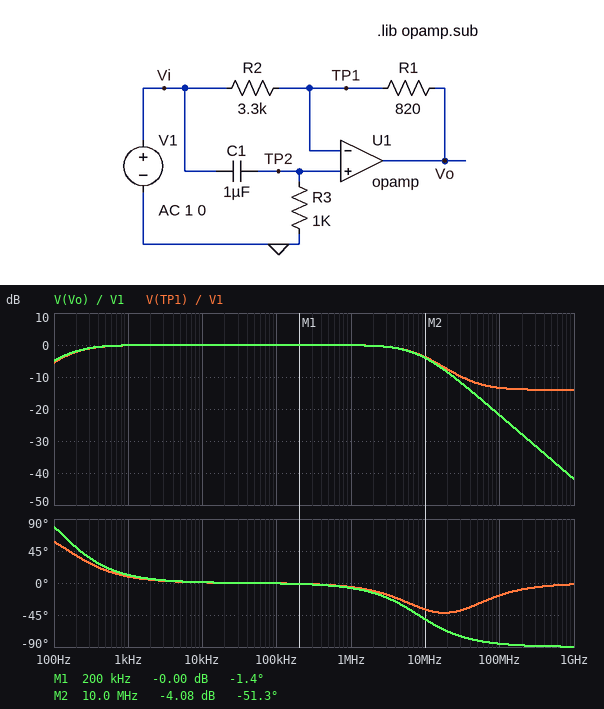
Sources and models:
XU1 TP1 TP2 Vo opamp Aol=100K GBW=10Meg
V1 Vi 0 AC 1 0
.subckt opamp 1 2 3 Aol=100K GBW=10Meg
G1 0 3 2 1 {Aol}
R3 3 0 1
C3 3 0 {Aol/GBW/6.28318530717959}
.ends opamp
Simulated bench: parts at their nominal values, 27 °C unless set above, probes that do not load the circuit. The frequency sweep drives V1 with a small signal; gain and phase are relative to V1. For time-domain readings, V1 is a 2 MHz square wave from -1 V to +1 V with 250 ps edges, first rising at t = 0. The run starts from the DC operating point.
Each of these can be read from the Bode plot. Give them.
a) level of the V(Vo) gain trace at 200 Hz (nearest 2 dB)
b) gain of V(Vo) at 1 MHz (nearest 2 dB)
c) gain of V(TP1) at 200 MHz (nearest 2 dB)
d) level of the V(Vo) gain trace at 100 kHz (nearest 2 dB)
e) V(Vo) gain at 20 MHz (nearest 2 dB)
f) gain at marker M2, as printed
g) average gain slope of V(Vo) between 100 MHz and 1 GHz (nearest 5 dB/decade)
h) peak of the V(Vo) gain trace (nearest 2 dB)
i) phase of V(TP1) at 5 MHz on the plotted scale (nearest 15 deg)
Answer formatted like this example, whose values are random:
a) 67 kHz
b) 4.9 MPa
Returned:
a) -2 dB
b) 0 dB
c) -14 dB
d) 0 dB
e) -8 dB
f) -4.08 dB
g) -20 dB/decade
h) 0 dB
i) -30 deg
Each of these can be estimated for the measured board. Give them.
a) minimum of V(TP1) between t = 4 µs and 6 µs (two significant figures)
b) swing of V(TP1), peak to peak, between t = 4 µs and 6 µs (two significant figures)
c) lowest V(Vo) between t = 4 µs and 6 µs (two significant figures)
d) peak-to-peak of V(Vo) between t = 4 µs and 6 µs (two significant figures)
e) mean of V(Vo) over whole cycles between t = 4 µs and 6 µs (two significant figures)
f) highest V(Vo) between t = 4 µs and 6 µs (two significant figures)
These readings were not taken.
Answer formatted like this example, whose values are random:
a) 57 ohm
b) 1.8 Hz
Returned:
a) -6.0 mV
b) 2.0 V
c) 240 mV
d) 2.0 V
e) 1.2 V
f) 2.2 V
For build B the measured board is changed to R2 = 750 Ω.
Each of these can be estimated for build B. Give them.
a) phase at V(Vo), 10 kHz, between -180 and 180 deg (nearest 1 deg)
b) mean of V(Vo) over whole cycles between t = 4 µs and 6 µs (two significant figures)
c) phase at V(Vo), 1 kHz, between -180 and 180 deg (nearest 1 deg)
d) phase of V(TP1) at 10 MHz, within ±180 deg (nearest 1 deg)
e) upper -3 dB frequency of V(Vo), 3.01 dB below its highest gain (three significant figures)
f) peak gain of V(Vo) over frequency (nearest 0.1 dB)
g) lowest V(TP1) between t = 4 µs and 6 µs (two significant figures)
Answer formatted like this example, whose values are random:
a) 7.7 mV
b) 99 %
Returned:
a) 2 deg
b) 2.1 V
c) 19 deg
d) -17 deg
e) 3.92 MHz
f) 0.8 dB
g) -5.5 mV
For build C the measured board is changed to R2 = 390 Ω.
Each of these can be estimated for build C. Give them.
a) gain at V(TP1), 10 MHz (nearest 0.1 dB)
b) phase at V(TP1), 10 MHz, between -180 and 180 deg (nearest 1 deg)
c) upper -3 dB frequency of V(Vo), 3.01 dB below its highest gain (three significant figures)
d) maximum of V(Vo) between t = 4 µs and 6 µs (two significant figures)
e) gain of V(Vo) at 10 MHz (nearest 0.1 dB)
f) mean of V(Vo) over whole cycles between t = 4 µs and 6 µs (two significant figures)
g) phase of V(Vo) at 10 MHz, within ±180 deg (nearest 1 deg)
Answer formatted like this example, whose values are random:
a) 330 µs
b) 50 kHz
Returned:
a) -2.9 dB
b) -8 deg
c) 215 Hz
d) 4.1 V
e) -10.3 dB
f) 3.1 V
g) -72 deg
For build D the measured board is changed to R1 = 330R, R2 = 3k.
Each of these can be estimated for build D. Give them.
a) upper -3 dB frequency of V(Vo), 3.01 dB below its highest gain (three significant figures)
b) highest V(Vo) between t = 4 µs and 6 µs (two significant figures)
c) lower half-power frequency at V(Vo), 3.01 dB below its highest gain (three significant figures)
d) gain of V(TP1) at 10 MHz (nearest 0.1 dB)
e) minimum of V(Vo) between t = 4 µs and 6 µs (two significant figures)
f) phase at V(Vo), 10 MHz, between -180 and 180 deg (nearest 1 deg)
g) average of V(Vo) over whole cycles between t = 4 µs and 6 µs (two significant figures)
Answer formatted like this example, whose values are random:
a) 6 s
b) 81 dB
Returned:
a) 9.01 MHz
b) 2.1 V
c) 157 Hz
d) -3.4 dB
e) 100 mV
f) -48 deg
g) 1.1 V
